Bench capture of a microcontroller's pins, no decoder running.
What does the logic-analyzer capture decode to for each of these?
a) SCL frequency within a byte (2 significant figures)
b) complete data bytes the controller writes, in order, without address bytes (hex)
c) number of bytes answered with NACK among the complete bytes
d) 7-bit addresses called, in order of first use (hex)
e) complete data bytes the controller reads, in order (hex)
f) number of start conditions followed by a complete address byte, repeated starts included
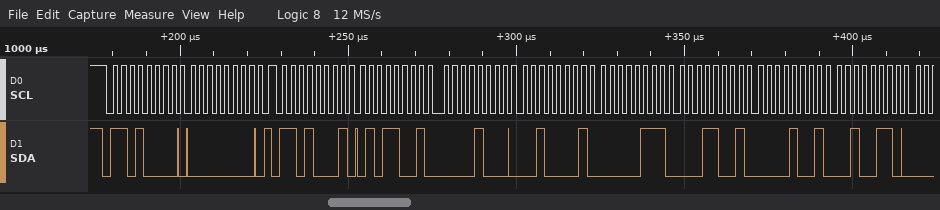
400 kHz
00
0
0x68
59 08 21 07 19 09 26
2
